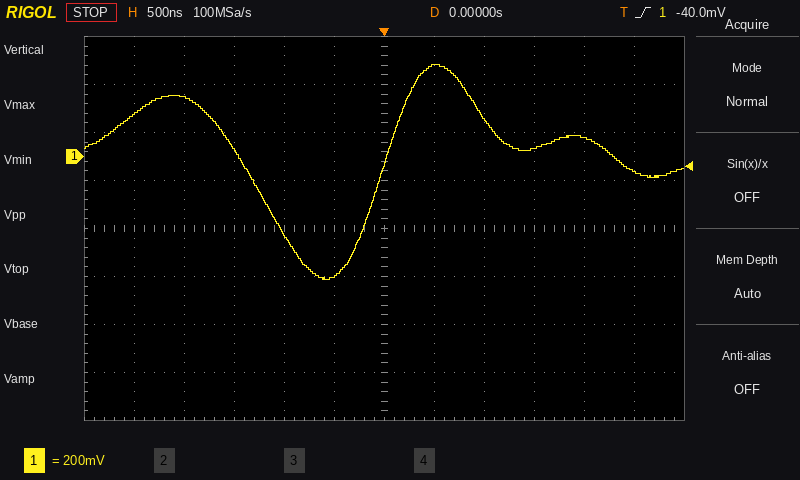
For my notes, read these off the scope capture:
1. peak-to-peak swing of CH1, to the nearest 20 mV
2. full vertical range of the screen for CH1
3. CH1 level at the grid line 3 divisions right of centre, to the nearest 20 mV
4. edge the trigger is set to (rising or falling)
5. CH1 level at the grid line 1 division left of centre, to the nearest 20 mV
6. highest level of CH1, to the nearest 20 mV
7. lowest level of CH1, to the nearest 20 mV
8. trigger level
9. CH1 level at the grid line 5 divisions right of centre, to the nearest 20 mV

900 mV
1.6 V
40 mV
rising
-500 mV
380 mV
-520 mV
-40.0 mV
-60 mV
